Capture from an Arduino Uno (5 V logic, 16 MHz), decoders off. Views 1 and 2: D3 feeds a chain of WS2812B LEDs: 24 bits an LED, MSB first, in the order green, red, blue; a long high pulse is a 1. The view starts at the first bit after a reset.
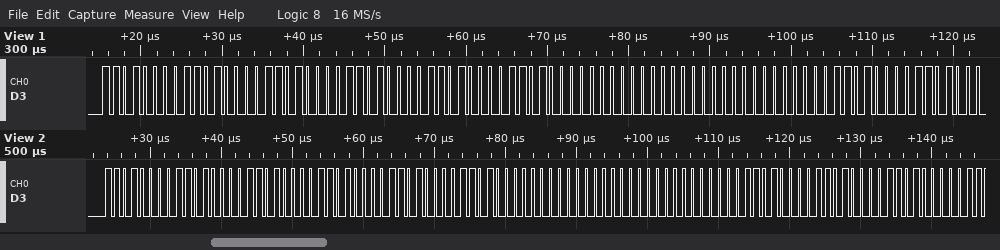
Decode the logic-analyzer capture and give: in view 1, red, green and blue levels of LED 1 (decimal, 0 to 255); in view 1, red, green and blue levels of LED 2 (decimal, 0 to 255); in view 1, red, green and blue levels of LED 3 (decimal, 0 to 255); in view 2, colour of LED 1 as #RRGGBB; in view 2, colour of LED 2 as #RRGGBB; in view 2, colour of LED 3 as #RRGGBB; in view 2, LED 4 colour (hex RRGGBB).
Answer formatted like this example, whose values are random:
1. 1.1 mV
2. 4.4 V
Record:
1. 208, 208, 208
2. 208, 208, 208
3. 0, 0, 0
4. #D0D0D0
5. #D0D0D0
6. #000000
7. #D0D0D0
